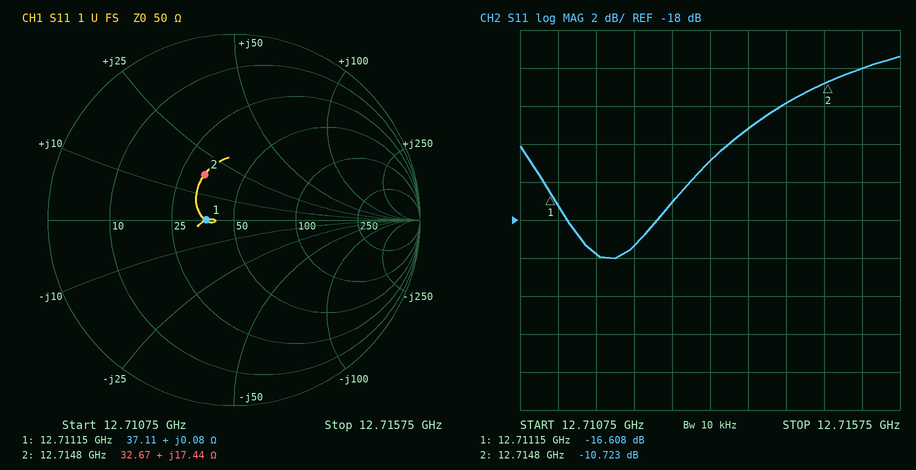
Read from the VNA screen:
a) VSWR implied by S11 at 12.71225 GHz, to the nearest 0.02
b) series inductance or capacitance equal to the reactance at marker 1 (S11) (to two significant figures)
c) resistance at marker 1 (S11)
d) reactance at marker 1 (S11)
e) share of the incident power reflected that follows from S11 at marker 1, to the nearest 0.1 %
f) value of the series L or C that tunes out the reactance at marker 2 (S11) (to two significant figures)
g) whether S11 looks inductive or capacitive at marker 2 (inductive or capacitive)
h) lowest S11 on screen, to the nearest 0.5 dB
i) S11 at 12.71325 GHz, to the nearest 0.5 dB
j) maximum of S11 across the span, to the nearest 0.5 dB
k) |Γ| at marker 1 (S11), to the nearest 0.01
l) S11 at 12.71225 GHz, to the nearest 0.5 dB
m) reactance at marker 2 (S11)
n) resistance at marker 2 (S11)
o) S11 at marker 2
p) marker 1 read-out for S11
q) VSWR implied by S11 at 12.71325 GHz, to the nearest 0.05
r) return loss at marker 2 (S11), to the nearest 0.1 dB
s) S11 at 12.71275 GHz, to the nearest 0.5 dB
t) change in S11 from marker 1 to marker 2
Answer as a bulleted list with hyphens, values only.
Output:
- 1.24
- 1.0 pH
- 37.11 Ω
- +0.08 Ω
- 2.2 %
- 720 fF
- inductive
- -20.0 dB
- -15.0 dB
- -9.5 dB
- 0.15
- -19.5 dB
- +17.44 Ω
- 32.67 Ω
- -10.723 dB
- -16.608 dB
- 1.45
- 10.7 dB
- -17.0 dB
- 5.885 dB
